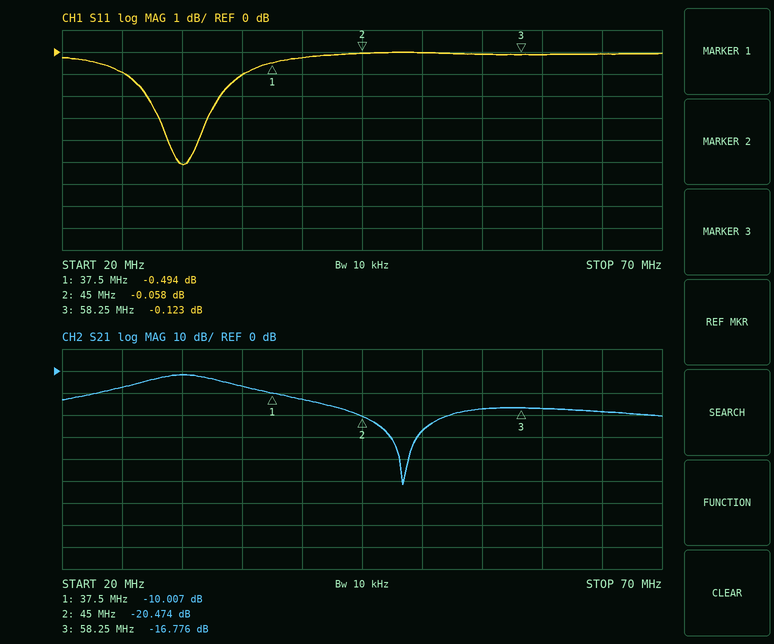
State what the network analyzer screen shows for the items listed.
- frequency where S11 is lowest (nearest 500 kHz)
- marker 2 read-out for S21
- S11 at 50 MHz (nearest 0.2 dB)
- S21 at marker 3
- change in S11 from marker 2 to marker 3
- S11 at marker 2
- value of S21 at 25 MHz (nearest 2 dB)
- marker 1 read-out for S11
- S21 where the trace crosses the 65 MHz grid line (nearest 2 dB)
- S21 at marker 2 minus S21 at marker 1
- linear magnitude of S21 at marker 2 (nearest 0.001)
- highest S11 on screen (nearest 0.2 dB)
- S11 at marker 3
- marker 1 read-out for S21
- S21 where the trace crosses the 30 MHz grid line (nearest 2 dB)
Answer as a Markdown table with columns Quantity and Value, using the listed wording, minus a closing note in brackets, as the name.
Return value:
| Quantity | Value |
|---|---|
| frequency where S11 is lowest | 30.0 MHz |
| marker 2 read-out for S21 | -20.474 dB |
| S11 at 50 MHz | 0.0 dB |
| S21 at marker 3 | -16.776 dB |
| change in S11 from marker 2 to marker 3 | -0.065 dB |
| S11 at marker 2 | -0.058 dB |
| value of S21 at 25 MHz | -8 dB |
| marker 1 read-out for S11 | -0.494 dB |
| S21 where the trace crosses the 65 MHz grid line | -18 dB |
| S21 at marker 2 minus S21 at marker 1 | -10.467 dB |
| linear magnitude of S21 at marker 2 | 0.095 |
| highest S11 on screen | 0.0 dB |
| S11 at marker 3 | -0.123 dB |
| marker 1 read-out for S21 | -10.007 dB |
| S21 where the trace crosses the 30 MHz grid line | -2 dB |
